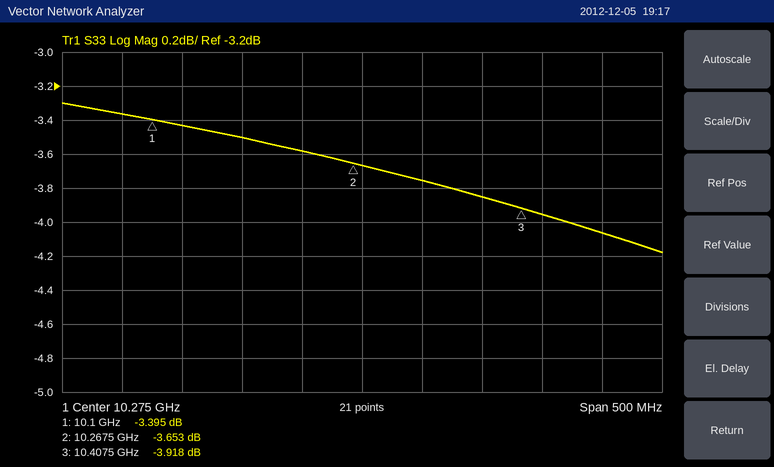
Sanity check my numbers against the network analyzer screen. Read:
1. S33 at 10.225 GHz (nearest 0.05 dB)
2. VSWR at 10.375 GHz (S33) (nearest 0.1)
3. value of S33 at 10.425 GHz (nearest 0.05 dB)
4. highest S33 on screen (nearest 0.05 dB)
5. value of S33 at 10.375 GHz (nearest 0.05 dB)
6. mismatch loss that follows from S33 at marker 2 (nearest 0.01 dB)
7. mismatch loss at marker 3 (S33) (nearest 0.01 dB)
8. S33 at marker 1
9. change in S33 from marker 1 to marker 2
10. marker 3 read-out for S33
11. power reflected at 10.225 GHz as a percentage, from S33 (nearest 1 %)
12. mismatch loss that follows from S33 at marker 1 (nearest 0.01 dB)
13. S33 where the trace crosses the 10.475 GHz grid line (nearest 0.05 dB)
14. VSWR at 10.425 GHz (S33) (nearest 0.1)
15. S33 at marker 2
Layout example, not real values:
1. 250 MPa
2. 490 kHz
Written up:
1. -3.60 dB
2. 4.6
3. -3.95 dB
4. -3.30 dB
5. -3.85 dB
6. 2.45 dB
7. 2.26 dB
8. -3.395 dB
9. -0.258 dB
10. -3.918 dB
11. 44 %
12. 2.66 dB
13. -4.05 dB
14. 4.5
15. -3.653 dB
